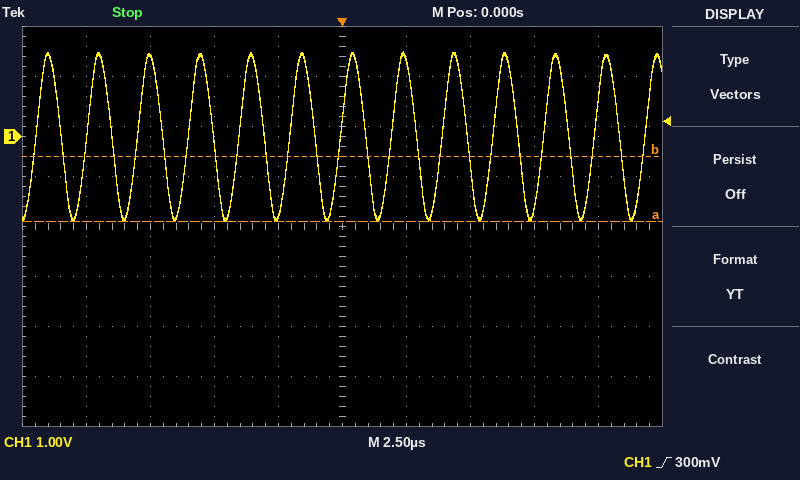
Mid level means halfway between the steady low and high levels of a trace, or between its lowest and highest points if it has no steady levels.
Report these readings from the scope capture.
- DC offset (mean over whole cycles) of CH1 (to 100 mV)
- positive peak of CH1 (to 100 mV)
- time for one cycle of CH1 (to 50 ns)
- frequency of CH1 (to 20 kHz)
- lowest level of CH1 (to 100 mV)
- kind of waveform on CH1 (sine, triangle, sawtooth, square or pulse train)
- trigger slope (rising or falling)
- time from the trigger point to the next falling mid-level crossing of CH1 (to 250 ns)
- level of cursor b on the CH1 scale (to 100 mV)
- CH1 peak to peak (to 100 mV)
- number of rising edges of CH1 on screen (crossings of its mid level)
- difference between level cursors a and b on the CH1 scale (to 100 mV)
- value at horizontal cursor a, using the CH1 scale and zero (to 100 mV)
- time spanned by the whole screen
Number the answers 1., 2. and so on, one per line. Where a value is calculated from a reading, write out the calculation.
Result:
1. (1.7 V + (-1.7 V)) / 2 ≈ 0.0 V
2. 1.7 V
3. 2.00 µs
4. 1 / 2.00 µs ≈ 500 kHz
5. -1.7 V
6. sine
7. rising
8. 1.00 µs
9. -400 mV
10. 1.7 V − (-1.7 V) = 3.4 V
11. 13
12. 1.3 V
13. -1.7 V
14. 25 µs
